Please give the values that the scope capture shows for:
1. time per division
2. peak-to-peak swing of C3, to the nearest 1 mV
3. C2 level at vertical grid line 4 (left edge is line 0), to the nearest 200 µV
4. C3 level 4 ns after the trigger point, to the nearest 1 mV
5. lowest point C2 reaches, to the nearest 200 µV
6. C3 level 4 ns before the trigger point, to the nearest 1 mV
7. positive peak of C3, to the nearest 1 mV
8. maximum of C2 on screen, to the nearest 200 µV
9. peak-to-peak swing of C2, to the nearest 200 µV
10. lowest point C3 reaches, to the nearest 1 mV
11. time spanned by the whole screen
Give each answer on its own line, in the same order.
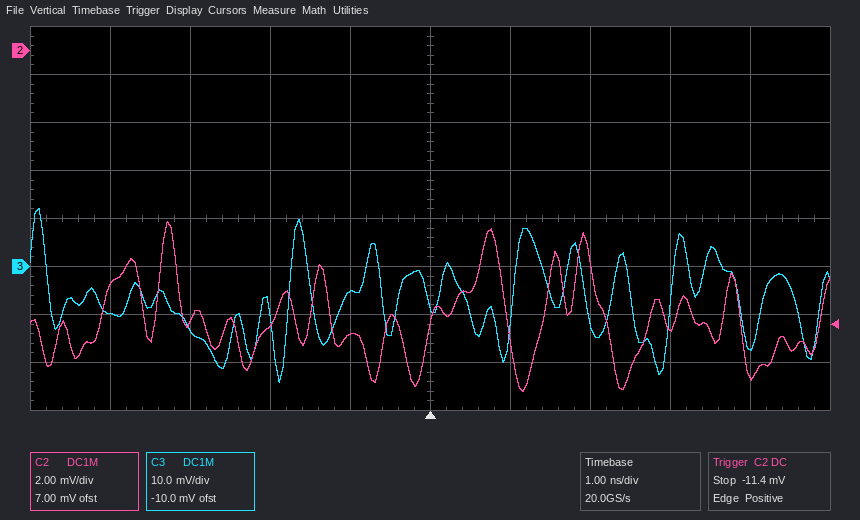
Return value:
1 ns
36 mV
-11.8 mV
-17 mV
-14.2 mV
-10 mV
12 mV
-7.2 mV
7.0 mV
-24 mV
10 ns
